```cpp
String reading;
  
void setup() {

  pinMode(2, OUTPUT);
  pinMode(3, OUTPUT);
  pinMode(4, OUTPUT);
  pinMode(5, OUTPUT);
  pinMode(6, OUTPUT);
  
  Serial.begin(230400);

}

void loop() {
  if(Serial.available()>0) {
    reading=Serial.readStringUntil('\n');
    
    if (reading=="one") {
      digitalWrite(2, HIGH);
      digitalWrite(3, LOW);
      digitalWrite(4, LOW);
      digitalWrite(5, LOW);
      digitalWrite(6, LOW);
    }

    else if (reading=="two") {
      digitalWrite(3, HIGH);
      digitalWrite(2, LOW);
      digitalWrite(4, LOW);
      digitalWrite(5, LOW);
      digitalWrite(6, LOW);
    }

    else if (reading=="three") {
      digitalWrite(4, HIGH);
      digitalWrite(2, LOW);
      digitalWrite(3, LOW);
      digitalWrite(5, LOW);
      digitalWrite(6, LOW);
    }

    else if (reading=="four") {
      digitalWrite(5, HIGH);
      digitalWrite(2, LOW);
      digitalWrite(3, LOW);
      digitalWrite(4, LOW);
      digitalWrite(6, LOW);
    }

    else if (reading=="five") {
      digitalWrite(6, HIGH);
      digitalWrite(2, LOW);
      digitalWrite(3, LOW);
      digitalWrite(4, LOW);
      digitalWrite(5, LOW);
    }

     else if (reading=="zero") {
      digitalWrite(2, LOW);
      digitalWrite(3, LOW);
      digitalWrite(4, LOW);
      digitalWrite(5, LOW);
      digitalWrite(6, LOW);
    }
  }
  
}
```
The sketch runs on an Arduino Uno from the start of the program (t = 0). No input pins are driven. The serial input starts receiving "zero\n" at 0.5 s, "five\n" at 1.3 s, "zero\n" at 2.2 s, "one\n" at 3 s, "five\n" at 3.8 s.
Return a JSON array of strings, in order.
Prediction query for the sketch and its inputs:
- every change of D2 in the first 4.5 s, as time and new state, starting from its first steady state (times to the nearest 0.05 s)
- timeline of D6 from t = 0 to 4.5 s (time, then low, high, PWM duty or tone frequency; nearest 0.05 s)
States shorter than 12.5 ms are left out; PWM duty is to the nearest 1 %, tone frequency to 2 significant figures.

["0 s low; 3 s high; 3.8 s low", "0 s low; 1.3 s high; 2.2 s low; 3.8 s high"]
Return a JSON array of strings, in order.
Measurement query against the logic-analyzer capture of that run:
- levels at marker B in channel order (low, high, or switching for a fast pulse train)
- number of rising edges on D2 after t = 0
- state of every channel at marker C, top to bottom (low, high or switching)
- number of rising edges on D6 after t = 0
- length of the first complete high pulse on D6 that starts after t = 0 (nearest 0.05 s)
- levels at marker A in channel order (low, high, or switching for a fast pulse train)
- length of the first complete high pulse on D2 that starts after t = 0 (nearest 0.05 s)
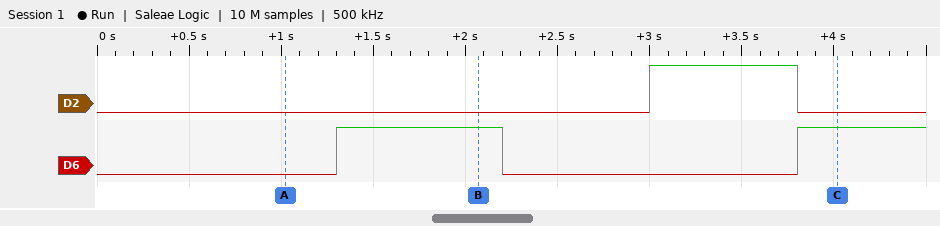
["D2 low, D6 high", "1", "D2 low, D6 high", "2", "0.90 s", "D2 low, D6 low", "0.80 s"]
